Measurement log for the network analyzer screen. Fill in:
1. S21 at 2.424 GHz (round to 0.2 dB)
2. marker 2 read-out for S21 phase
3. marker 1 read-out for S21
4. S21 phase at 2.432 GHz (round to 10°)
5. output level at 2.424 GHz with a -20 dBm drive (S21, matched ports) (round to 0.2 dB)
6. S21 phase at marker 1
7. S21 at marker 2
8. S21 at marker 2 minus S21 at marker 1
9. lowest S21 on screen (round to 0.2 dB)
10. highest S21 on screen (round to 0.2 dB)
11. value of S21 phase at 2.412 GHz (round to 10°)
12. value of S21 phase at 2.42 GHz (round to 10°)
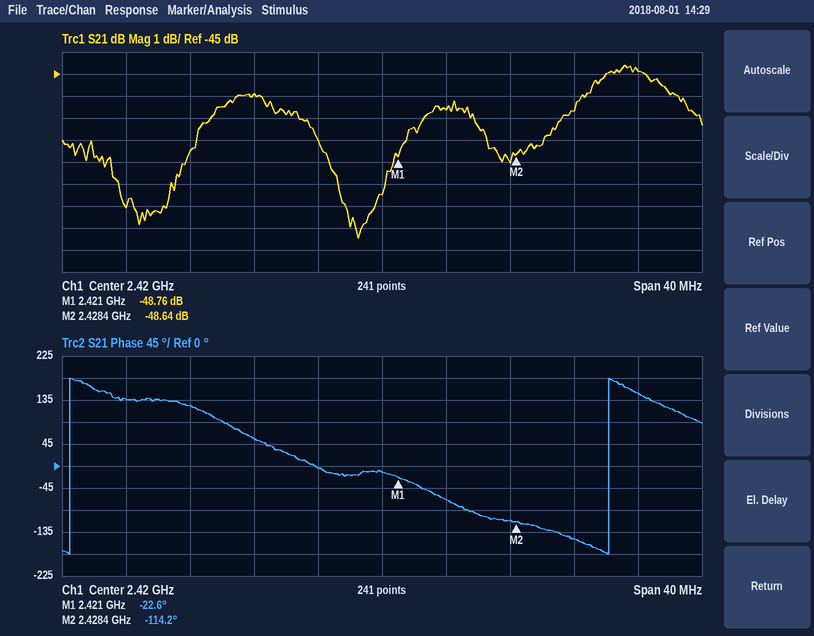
-46.6 dB
-114.2°
-48.76 dB
-150°
-66.6 dBm
-22.6°
-48.64 dB
0.12 dB
-52.4 dB
-44.6 dB
60°
-10°
